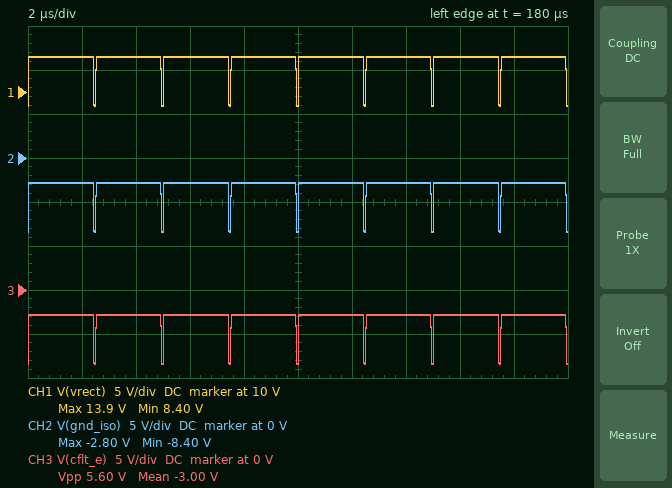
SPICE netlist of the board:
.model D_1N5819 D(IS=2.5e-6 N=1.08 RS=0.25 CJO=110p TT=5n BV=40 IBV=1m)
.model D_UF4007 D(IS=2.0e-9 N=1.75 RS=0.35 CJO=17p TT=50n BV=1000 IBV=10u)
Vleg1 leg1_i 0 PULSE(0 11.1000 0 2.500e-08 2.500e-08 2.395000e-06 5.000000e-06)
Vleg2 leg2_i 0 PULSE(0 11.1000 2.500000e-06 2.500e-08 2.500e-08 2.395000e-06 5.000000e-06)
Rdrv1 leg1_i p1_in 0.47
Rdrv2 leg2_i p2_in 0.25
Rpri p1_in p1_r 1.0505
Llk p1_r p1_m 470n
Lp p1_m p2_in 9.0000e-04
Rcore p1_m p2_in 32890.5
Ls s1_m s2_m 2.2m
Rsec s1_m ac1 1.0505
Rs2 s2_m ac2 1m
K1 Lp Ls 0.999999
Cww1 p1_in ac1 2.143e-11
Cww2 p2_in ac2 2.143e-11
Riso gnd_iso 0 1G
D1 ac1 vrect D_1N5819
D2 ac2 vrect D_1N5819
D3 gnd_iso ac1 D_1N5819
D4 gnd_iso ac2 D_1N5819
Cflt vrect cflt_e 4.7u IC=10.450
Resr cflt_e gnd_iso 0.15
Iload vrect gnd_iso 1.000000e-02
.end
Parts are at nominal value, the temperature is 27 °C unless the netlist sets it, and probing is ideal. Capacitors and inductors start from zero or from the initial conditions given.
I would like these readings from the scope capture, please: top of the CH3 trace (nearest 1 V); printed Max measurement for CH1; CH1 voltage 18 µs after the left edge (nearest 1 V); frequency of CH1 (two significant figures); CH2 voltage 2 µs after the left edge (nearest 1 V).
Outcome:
-3 V
13.9 V
14 V
400 kHz
-3 V
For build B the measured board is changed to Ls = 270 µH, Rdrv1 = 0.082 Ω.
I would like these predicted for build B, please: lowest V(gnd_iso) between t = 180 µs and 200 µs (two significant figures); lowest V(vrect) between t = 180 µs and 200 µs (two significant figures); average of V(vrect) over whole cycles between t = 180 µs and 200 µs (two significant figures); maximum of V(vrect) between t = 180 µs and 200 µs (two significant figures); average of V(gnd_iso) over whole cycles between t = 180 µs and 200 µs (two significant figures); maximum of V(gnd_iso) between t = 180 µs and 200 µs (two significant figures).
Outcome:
-5.0 V
5.0 V
10 V
11 V
350 mV
540 mV
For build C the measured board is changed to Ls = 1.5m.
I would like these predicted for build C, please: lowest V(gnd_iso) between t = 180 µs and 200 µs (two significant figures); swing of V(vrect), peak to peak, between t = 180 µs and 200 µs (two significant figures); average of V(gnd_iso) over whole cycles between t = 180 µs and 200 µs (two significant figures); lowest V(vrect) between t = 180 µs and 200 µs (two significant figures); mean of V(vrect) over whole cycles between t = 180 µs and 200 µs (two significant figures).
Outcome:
-6.9 V
5.6 V
-1.5 V
6.9 V
12 V
